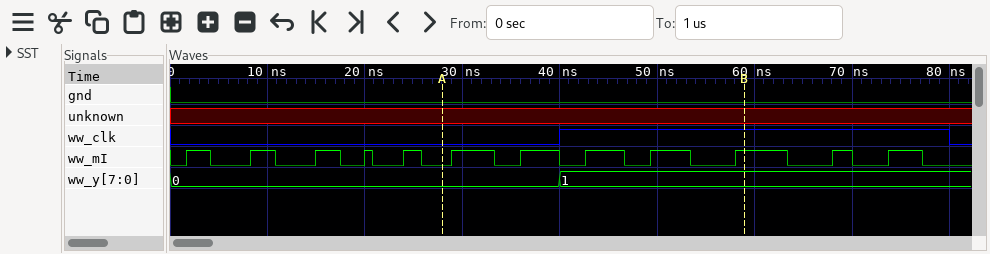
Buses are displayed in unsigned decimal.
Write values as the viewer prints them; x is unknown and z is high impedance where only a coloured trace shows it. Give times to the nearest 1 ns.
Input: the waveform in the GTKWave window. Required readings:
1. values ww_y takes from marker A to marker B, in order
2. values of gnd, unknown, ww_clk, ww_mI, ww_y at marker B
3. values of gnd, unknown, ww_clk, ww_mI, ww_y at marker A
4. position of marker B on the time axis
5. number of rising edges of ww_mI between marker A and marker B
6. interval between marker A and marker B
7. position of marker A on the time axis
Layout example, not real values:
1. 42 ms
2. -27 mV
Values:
1. 0, 1
2. gnd=0, unknown=x, ww_clk=1, ww_mI=1, ww_y=1
3. gnd=0, unknown=x, ww_clk=0, ww_mI=0, ww_y=0
4. 59 ns
5. 5
6. 31 ns
7. 28 ns
